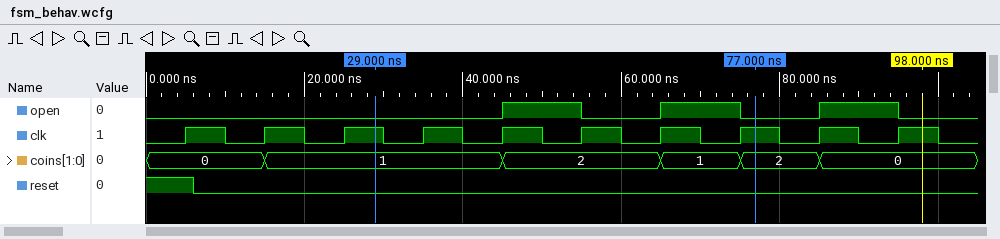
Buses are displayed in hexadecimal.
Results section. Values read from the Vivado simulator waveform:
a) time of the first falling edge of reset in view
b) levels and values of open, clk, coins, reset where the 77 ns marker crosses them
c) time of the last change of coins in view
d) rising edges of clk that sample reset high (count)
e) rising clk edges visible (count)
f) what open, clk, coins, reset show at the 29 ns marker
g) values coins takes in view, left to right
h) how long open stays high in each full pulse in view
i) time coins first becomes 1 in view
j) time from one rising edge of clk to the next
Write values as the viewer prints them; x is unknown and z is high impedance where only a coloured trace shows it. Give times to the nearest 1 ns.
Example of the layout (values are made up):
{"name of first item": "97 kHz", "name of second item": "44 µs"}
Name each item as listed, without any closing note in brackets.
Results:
{"time of the first falling edge of reset in view": "6 ns", "levels and values of open, clk, coins, reset where the 77 ns marker crosses them": "open=0, clk=1, coins=2, reset=0", "time of the last change of coins in view": "85 ns", "rising edges of clk that sample reset high": "1", "rising clk edges visible": "10", "what open, clk, coins, reset show at the 29 ns marker": "open=0, clk=1, coins=1, reset=0", "values coins takes in view, left to right": "0, 1, 2, 1, 2, 0", "how long open stays high in each full pulse in view": "10 ns, 10 ns, 10 ns", "time coins first becomes 1 in view": "15 ns", "time from one rising edge of clk to the next": "10 ns"}
